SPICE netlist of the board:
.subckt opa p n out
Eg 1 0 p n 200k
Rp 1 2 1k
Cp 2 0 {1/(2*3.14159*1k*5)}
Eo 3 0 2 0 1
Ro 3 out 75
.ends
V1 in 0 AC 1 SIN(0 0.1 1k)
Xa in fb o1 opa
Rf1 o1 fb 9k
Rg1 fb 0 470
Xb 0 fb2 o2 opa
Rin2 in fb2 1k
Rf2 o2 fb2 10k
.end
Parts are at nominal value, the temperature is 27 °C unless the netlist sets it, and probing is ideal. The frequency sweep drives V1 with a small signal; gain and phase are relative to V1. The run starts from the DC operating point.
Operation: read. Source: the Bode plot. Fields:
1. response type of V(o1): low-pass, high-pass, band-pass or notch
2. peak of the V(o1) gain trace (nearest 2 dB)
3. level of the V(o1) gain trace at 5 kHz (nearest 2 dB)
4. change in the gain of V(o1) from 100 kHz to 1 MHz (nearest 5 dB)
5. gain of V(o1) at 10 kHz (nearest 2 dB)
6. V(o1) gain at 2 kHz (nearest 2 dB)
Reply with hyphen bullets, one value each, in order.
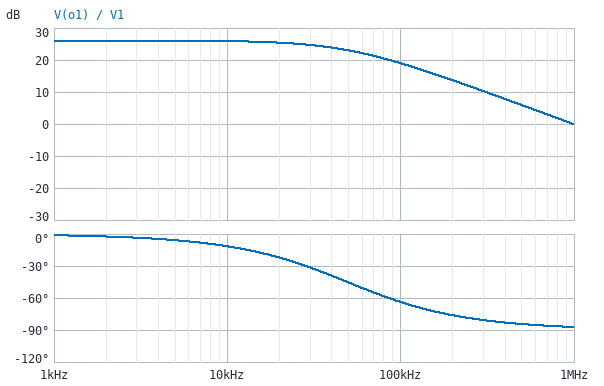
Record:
- low-pass
- 26 dB
- 26 dB
- -20 dB
- 26 dB
- 26 dB
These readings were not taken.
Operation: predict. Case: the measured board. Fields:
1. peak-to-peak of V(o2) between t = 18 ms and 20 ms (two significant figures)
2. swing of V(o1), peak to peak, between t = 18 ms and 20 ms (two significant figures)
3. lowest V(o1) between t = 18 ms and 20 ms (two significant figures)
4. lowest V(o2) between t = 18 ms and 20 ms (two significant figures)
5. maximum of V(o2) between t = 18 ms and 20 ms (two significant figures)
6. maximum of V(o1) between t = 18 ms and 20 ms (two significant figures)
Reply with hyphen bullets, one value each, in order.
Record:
- 2.0 V
- 4.0 V
- -2.0 V
- -1.0 V
- 1.0 V
- 2.0 V
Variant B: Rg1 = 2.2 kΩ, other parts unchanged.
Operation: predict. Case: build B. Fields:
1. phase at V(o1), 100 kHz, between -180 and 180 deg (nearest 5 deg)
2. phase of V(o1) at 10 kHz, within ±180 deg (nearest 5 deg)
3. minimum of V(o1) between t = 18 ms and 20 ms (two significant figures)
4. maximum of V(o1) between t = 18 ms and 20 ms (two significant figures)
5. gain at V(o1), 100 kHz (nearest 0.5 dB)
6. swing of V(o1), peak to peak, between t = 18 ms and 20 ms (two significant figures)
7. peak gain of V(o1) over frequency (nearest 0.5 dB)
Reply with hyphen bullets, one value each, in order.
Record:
- -25 deg
- -5 deg
- -510 mV
- 510 mV
- 13.0 dB
- 1.0 V
- 14.0 dB
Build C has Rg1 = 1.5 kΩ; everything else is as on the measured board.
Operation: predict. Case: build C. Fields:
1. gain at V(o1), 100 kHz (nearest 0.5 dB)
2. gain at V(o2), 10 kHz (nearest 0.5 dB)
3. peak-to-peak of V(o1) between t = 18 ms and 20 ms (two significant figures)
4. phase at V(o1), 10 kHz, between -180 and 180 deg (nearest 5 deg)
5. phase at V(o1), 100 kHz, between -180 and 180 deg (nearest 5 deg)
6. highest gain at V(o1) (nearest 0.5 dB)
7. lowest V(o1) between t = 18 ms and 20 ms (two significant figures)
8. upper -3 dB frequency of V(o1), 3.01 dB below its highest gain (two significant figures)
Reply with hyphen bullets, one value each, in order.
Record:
- 15.0 dB
- 20.0 dB
- 1.4 V
- -5 deg
- -35 deg
- 17.0 dB
- -700 mV
- 140 kHz
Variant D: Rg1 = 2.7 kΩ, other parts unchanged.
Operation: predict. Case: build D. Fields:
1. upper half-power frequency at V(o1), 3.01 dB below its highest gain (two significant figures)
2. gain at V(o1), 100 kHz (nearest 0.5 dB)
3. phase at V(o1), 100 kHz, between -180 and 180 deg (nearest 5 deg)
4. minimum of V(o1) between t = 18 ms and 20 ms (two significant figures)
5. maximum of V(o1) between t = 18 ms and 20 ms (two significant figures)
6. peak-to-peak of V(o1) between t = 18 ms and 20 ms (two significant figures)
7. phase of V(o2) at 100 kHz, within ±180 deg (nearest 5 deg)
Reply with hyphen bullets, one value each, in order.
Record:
- 230 kHz
- 12.0 dB
- -25 deg
- -430 mV
- 430 mV
- 870 mV
- 130 deg
